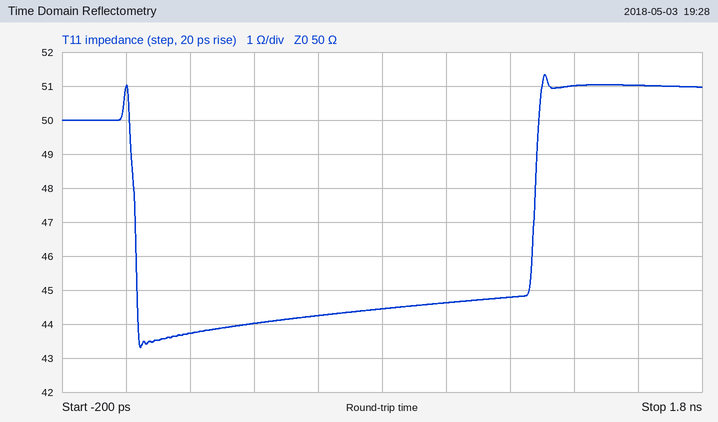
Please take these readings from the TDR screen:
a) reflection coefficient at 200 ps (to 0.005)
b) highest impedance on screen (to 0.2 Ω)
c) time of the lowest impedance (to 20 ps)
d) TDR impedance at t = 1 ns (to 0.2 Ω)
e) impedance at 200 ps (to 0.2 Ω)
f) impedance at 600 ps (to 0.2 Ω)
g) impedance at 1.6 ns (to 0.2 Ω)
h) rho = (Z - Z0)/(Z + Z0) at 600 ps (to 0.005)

-0.065
51.4 Ω
40 ps
44.6 Ω
43.8 Ω
44.2 Ω
51.0 Ω
-0.060
